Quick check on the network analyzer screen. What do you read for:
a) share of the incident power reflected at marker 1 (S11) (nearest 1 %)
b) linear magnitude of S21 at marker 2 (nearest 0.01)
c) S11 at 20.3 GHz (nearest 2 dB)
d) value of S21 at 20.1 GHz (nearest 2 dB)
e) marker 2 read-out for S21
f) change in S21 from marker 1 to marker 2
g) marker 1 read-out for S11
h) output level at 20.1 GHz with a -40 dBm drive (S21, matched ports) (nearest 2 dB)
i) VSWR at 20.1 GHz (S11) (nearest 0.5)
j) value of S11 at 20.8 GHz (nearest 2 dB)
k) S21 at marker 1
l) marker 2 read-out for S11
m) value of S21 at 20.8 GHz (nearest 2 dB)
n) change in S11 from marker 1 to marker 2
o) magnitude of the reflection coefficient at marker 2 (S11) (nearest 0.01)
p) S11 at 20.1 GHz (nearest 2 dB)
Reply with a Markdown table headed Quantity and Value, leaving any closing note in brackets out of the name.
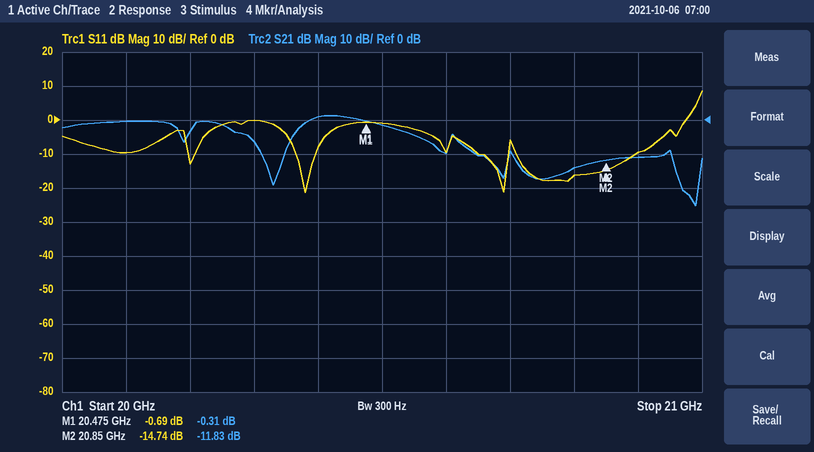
| Quantity | Value |
|---|---|
| share of the incident power reflected at marker 1 (S11) | 85 % |
| linear magnitude of S21 at marker 2 | 0.26 |
| S11 at 20.3 GHz | 0 dB |
| value of S21 at 20.1 GHz | 0 dB |
| marker 2 read-out for S21 | -11.83 dB |
| change in S21 from marker 1 to marker 2 | -11.52 dB |
| marker 1 read-out for S11 | -0.69 dB |
| output level at 20.1 GHz with a -40 dBm drive (S21, matched ports) | -40 dBm |
| VSWR at 20.1 GHz (S11) | 2.0 |
| value of S11 at 20.8 GHz | -16 dB |
| S21 at marker 1 | -0.31 dB |
| marker 2 read-out for S11 | -14.74 dB |
| value of S21 at 20.8 GHz | -14 dB |
| change in S11 from marker 1 to marker 2 | -14.05 dB |
| magnitude of the reflection coefficient at marker 2 (S11) | 0.18 |
| S11 at 20.1 GHz | -10 dB |
